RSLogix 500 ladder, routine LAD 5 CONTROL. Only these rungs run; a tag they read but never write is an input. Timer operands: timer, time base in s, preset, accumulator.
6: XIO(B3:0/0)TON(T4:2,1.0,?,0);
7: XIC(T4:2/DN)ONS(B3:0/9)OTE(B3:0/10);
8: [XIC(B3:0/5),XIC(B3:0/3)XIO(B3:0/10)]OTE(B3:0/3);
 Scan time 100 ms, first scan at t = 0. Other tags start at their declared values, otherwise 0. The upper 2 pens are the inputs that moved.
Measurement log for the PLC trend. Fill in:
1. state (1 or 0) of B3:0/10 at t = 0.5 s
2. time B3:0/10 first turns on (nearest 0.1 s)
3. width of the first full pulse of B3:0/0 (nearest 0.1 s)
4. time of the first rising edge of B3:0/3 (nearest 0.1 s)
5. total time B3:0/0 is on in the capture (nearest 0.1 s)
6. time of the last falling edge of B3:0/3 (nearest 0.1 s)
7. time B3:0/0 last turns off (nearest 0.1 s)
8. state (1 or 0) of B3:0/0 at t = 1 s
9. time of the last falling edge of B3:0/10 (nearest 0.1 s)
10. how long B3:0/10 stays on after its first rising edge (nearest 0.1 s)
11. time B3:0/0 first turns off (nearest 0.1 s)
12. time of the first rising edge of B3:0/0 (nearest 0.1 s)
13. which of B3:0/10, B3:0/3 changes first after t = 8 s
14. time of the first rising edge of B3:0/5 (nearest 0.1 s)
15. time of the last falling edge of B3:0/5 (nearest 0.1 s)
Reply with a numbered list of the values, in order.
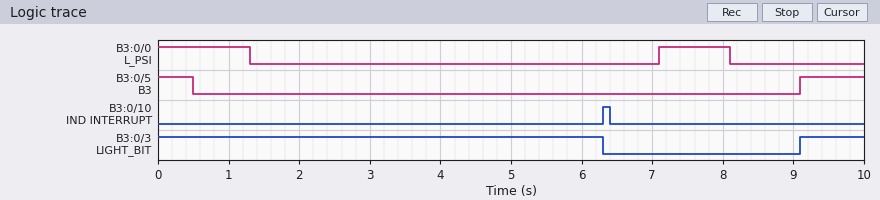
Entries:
1. 0
2. 6.3 s
3. 1.0 s
4. 9.1 s
5. 2.3 s
6. 6.3 s
7. 8.1 s
8. 1
9. 6.4 s
10. 0.1 s
11. 1.3 s
12. 7.1 s
13. B3:0/3
14. 9.1 s
15. 0.5 s
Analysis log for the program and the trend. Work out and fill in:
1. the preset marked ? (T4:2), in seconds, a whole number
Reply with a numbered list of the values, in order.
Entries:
1. 5 s
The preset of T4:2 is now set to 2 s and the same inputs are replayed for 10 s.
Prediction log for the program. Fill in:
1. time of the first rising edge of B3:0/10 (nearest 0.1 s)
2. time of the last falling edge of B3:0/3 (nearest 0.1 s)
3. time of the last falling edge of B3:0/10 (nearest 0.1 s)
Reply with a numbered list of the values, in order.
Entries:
1. 3.3 s
2. 3.3 s
3. 3.4 s
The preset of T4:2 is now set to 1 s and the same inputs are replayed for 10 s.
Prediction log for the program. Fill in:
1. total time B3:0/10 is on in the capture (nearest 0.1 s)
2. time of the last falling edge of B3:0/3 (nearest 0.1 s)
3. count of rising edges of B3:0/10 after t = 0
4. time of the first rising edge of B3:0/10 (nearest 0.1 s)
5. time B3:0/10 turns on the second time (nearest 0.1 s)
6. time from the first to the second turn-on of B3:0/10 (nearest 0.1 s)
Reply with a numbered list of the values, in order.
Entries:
1. 0.2 s
2. 2.3 s
3. 2
4. 2.3 s
5. 9.1 s
6. 6.8 s
